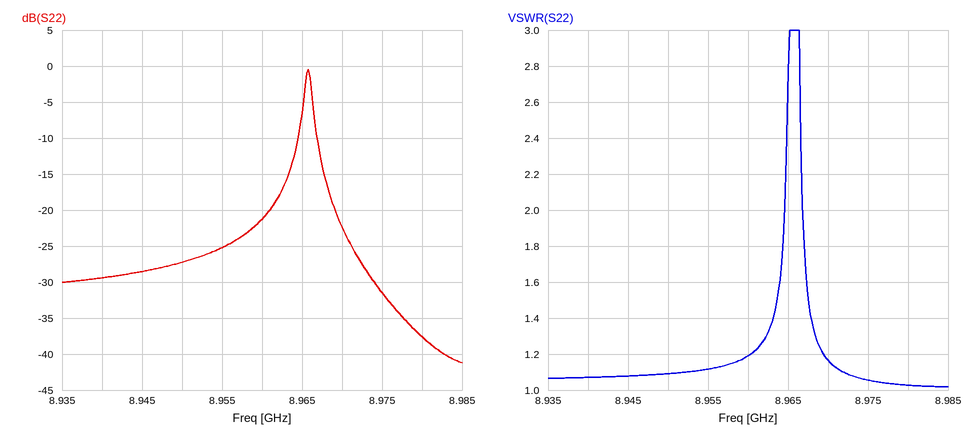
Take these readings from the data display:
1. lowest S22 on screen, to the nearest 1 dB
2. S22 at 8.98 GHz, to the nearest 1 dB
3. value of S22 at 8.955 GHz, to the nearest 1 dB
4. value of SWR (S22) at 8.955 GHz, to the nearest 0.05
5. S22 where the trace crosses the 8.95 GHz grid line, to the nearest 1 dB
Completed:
-41 dB
-38 dB
-25 dB
1.10
-27 dB
